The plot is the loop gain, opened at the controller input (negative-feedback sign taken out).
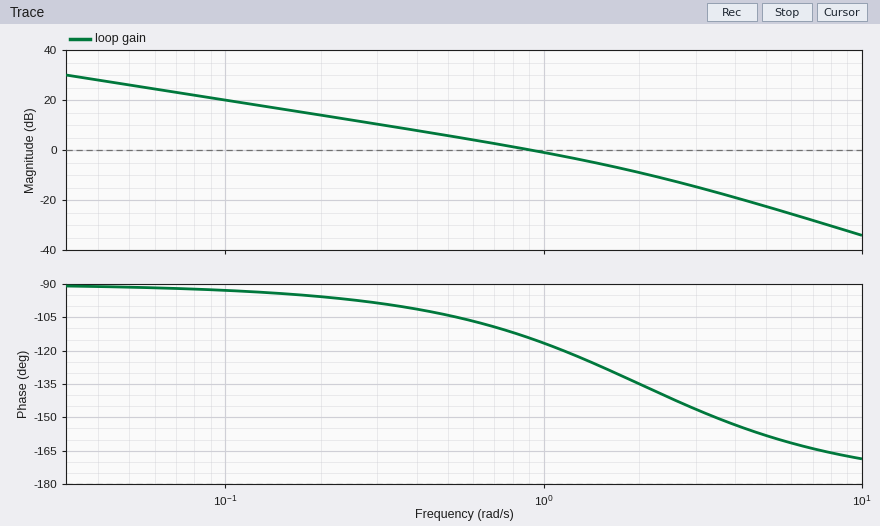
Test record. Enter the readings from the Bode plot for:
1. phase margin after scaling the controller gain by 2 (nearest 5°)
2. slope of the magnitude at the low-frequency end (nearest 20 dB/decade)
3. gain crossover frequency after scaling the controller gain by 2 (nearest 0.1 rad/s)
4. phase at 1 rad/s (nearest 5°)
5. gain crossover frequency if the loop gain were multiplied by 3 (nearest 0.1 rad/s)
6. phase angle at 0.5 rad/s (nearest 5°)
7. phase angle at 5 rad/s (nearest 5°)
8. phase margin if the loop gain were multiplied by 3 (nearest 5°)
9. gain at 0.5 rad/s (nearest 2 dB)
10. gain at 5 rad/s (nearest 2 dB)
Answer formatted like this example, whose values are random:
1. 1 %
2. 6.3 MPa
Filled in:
1. 50°
2. -20 dB/decade
3. 1.6 rad/s
4. -115°
5. 2.1 rad/s
6. -105°
7. -160°
8. 45°
9. 6 dB
10. -22 dB
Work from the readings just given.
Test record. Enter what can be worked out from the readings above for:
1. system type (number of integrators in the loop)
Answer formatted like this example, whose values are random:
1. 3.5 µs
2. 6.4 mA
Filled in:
1. 1
